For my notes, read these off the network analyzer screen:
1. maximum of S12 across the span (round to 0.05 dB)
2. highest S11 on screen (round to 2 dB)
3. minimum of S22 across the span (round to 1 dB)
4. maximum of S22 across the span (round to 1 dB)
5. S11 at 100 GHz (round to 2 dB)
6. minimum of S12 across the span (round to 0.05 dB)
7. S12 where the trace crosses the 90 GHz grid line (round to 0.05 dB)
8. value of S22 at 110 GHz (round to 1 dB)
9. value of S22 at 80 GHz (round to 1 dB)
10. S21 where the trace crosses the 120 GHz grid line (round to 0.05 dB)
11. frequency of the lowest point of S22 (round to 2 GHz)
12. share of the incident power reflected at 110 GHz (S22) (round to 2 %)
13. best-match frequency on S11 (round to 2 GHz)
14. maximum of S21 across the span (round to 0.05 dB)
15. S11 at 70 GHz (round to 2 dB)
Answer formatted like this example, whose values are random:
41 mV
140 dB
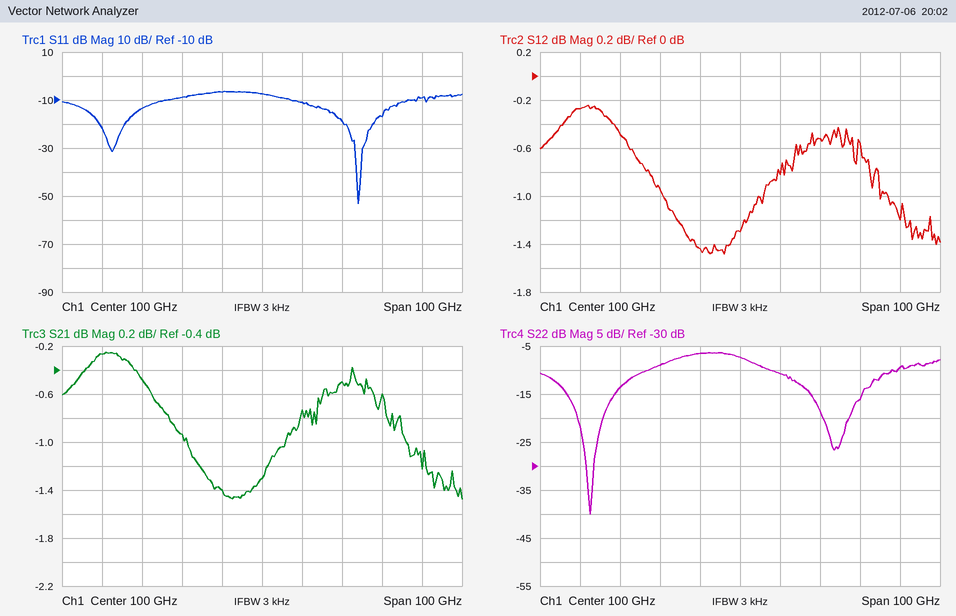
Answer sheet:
-0.25 dB
-6 dB
-40 dB
-6 dB
-8 dB
-1.50 dB
-1.45 dB
-11 dB
-9 dB
-0.50 dB
62 GHz
8 %
124 GHz
-0.25 dB
-14 dB
